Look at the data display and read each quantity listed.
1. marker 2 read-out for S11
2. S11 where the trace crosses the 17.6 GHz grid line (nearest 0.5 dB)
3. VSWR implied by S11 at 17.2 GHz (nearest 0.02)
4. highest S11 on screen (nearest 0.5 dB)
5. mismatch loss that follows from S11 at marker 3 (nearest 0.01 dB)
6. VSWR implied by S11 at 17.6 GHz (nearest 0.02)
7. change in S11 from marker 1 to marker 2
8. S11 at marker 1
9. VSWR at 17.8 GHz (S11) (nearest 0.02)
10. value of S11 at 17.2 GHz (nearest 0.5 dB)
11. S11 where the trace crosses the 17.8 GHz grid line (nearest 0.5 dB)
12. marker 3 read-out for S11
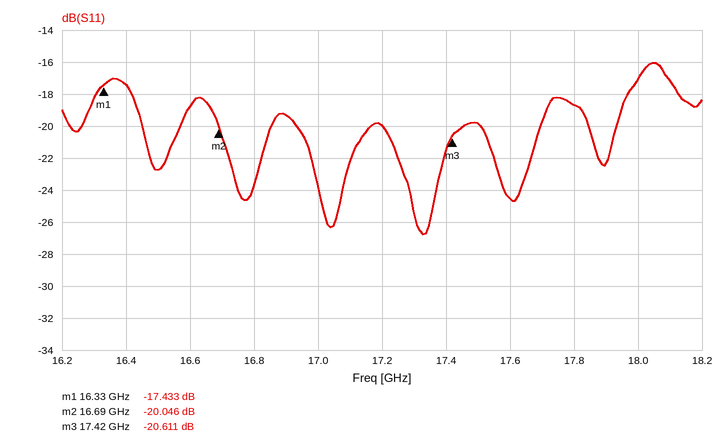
-20.046 dB
-24.5 dB
1.22
-16.0 dB
0.04 dB
1.12
-2.613 dB
-17.433 dB
1.26
-20.0 dB
-18.5 dB
-20.611 dB
